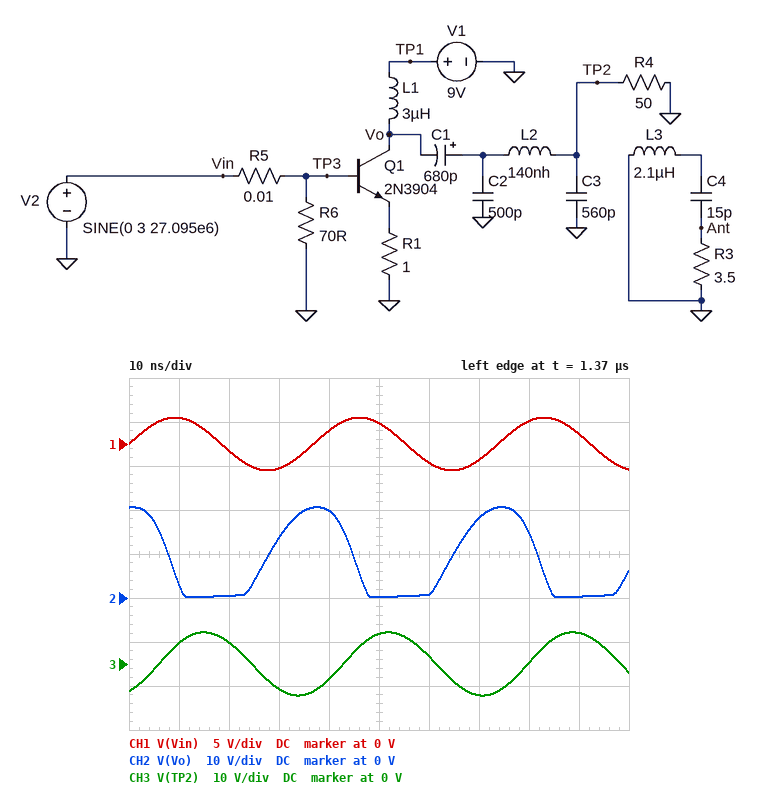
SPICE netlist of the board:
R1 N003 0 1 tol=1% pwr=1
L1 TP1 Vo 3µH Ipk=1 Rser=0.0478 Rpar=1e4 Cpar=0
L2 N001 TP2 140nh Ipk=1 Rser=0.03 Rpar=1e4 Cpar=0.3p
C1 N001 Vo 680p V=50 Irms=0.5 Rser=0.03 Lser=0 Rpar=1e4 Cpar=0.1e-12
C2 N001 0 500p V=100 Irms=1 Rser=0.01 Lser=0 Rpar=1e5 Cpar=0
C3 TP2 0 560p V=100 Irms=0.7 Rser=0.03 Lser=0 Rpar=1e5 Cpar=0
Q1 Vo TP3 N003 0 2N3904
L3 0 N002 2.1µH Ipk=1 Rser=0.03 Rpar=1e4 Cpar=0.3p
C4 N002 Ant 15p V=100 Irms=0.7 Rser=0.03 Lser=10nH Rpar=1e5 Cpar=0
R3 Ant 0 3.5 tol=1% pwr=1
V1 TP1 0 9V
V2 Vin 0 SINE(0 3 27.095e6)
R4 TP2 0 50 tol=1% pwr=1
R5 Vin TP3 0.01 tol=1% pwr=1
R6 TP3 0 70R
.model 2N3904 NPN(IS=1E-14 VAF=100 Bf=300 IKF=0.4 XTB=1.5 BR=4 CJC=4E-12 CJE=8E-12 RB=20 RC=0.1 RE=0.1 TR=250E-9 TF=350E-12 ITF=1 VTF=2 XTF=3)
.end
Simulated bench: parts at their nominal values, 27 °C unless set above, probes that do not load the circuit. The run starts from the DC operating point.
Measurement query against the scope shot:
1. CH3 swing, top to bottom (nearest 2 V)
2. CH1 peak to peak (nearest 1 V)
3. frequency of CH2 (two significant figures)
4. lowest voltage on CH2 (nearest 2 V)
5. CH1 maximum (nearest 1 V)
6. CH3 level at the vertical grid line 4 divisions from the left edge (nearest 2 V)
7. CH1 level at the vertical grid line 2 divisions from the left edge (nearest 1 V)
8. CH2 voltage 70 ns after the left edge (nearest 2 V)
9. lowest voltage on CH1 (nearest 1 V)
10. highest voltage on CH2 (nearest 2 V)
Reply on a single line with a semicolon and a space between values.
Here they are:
14 V; 6 V; 27 MHz; 0 V; 3 V; -4 V; -1 V; 18 V; -3 V; 20 V
